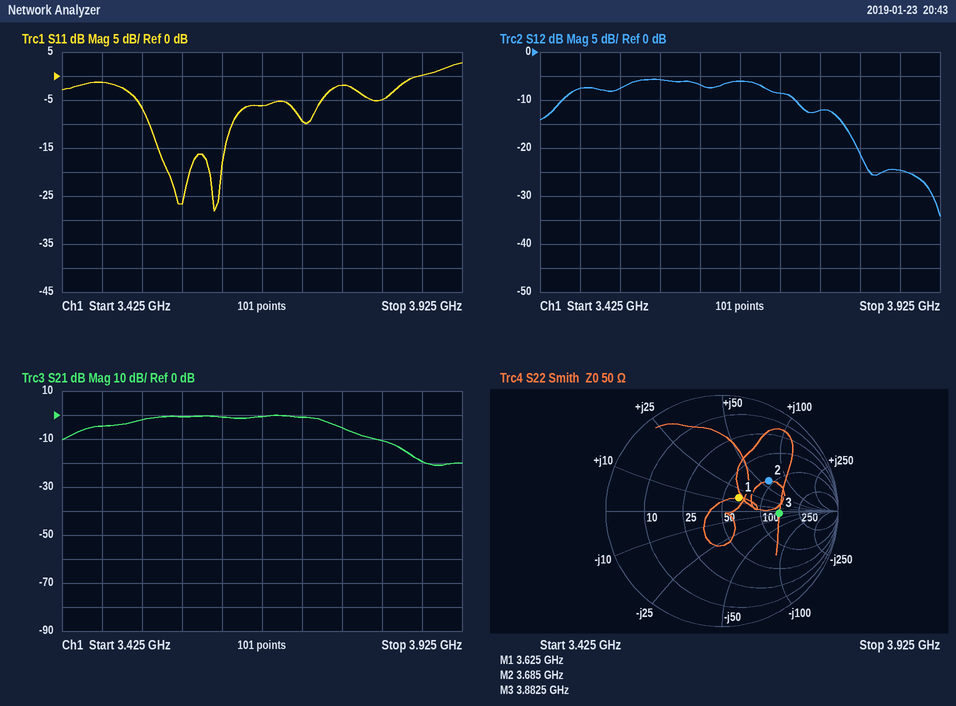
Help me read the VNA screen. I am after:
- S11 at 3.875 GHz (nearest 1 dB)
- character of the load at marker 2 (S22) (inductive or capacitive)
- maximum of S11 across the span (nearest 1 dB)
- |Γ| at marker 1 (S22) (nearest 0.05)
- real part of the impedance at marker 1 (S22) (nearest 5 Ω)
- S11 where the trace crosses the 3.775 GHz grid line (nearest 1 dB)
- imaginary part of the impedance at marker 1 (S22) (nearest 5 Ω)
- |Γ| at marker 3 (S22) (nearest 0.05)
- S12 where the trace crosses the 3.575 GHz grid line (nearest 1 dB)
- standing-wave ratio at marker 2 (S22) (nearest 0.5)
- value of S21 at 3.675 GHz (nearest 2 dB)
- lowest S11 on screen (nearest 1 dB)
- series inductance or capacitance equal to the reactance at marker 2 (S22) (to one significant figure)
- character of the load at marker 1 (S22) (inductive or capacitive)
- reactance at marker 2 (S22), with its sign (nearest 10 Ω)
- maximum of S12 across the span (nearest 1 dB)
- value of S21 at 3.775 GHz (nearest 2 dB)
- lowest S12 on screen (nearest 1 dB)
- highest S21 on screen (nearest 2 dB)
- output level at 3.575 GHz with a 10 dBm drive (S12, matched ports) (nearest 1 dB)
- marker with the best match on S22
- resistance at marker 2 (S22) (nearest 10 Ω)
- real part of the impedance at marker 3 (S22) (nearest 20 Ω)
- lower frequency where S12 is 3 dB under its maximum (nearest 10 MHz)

0 dB
inductive
3 dB
0.20
65 Ω
-2 dB
+15 Ω
0.50
-6 dB
3.0
0 dB
-28 dB
3 nH
inductive
+60 Ω
-6 dB
-6 dB
-34 dB
0 dB
4 dBm
marker 1
90 Ω
140 Ω
3.46 GHz
